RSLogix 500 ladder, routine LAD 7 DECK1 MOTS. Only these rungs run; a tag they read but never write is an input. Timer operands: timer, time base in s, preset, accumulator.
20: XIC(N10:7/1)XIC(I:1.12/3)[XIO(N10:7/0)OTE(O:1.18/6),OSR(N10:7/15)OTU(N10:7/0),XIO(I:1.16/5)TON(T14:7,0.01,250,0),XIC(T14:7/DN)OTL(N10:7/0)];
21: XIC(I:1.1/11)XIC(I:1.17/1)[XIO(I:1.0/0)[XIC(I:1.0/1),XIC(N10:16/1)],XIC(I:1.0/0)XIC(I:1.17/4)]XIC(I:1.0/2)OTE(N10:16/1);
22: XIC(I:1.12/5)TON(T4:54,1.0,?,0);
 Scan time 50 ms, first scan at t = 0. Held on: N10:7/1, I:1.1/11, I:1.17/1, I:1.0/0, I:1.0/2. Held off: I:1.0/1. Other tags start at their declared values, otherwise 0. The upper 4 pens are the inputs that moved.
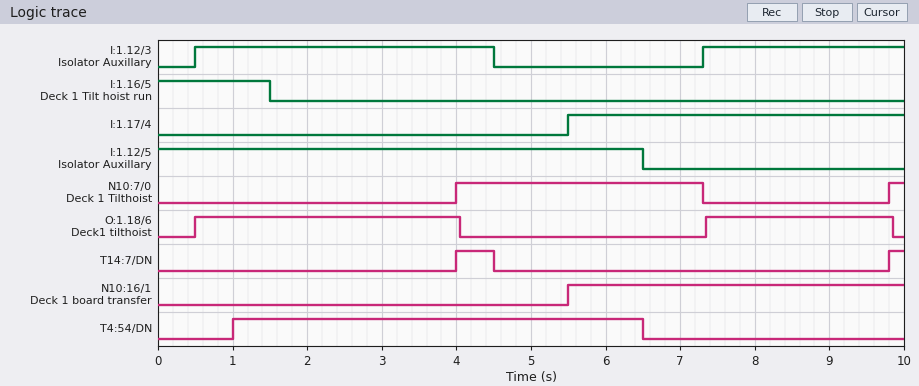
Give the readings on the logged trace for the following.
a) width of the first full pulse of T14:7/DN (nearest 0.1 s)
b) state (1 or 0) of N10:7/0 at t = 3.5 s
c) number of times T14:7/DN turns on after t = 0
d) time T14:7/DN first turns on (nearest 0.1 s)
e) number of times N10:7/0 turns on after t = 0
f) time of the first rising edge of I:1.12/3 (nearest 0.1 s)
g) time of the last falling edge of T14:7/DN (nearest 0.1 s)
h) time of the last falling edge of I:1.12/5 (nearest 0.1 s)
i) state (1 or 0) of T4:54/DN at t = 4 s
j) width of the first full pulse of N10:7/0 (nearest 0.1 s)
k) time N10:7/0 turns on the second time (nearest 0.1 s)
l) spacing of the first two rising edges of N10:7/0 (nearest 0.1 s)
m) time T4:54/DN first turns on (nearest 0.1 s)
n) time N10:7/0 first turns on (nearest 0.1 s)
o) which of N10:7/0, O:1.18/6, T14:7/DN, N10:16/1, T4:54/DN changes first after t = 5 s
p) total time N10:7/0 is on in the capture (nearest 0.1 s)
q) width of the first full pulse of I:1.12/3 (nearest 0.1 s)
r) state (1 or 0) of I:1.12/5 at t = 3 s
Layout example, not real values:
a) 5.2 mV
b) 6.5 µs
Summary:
a) 0.5 s
b) 0
c) 2
d) 4.0 s
e) 2
f) 0.5 s
g) 4.5 s
h) 6.5 s
i) 1
j) 3.3 s
k) 9.8 s
l) 5.8 s
m) 1.0 s
n) 4.0 s
o) N10:16/1
p) 3.5 s
q) 4.0 s
r) 1
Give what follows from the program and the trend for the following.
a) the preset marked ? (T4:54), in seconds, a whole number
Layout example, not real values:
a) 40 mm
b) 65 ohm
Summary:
a) 1 s
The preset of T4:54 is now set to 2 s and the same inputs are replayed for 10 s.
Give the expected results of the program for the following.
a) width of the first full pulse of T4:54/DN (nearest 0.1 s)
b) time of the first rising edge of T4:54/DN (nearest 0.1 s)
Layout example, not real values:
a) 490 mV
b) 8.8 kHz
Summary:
a) 4.5 s
b) 2.0 s
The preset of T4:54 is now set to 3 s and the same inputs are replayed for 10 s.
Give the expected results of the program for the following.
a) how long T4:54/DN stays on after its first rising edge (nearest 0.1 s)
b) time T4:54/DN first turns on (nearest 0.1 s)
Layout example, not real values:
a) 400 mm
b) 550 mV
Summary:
a) 3.5 s
b) 3.0 s
